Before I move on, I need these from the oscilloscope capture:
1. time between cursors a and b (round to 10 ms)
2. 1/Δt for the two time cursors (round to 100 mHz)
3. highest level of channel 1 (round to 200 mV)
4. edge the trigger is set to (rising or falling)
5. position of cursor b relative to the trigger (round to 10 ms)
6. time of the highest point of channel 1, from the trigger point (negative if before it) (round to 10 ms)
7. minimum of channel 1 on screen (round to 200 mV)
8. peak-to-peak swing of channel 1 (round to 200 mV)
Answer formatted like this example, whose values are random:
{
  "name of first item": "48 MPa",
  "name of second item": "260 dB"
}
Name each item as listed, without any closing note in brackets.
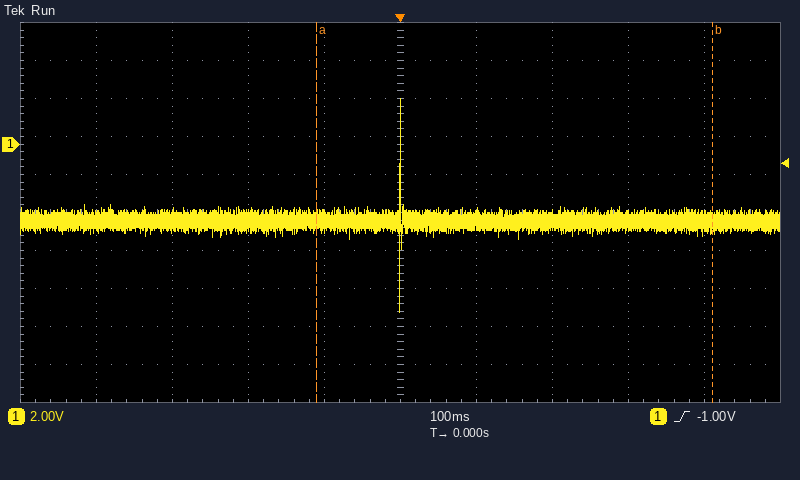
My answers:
{
  "time between cursors a and b": "520 ms",
  "1/Δt for the two time cursors": "1.9 Hz",
  "highest level of channel 1": "2.4 V",
  "edge the trigger is set to": "rising",
  "position of cursor b relative to the trigger": "+410 ms",
  "time of the highest point of channel 1, from the trigger point (negative if before it)": "0 ms",
  "minimum of channel 1 on screen": "-8.8 V",
  "peak-to-peak swing of channel 1": "11.2 V"
}
